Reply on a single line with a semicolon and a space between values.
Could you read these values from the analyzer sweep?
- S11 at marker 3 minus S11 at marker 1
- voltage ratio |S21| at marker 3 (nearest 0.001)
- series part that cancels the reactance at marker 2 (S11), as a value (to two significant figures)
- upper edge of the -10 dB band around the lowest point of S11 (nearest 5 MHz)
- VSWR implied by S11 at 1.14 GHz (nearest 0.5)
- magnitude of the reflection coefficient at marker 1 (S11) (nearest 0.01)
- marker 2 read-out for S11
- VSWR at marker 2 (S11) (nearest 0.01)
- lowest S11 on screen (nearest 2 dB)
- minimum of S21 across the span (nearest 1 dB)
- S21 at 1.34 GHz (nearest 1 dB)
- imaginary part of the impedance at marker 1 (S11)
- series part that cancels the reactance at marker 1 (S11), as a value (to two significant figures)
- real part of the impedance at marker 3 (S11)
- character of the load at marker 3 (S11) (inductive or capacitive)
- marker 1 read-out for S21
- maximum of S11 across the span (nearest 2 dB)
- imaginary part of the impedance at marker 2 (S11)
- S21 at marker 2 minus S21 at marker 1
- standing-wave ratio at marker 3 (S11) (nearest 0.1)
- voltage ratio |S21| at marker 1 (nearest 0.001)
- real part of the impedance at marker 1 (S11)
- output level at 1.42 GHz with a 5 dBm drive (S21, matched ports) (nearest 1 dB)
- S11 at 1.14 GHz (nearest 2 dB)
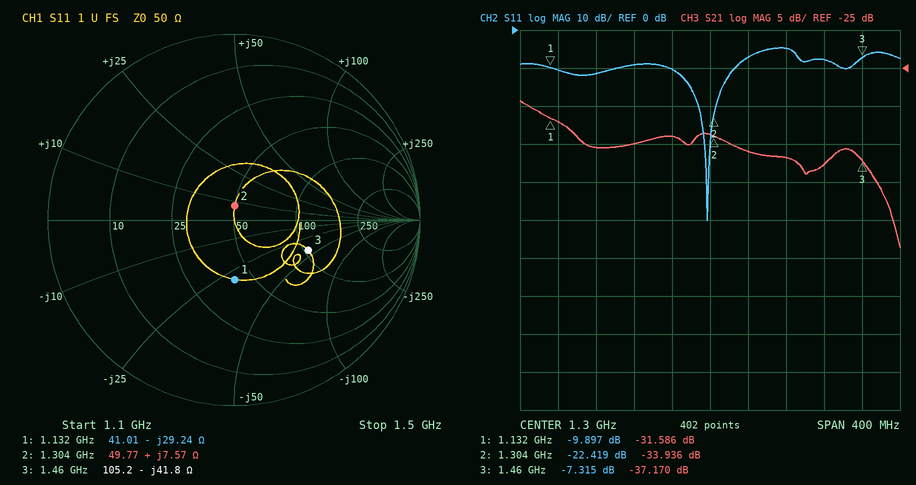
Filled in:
2.582 dB; 0.014; 16 pF; 1.325 GHz; 2.0; 0.32; -22.419 dB; 1.16; -50 dB; -49 dB; -36 dB; -29.24 Ω; 4.1 nH; 105.2 Ω; capacitive; -31.586 dB; -4 dB; +7.57 Ω; -2.350 dB; 2.5; 0.026; 41.01 Ω; -33 dBm; -10 dB
